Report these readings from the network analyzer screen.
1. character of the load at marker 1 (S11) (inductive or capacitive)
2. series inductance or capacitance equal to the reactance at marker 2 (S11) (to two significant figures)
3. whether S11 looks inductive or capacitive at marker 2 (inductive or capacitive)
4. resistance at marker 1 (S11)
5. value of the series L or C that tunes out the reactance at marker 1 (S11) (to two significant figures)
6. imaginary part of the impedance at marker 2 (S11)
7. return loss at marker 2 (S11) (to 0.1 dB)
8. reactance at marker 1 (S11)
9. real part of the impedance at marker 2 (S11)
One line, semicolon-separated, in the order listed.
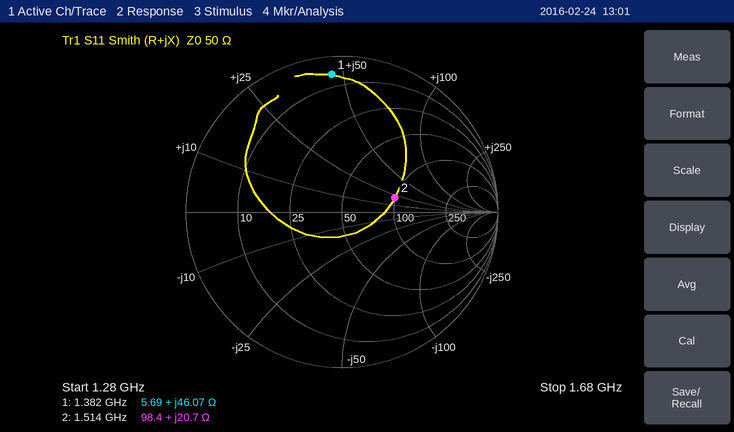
inductive; 2.2 nH; inductive; 5.69 Ω; 2.5 pF; +20.7 Ω; 9.1 dB; +46.07 Ω; 98.4 Ω
